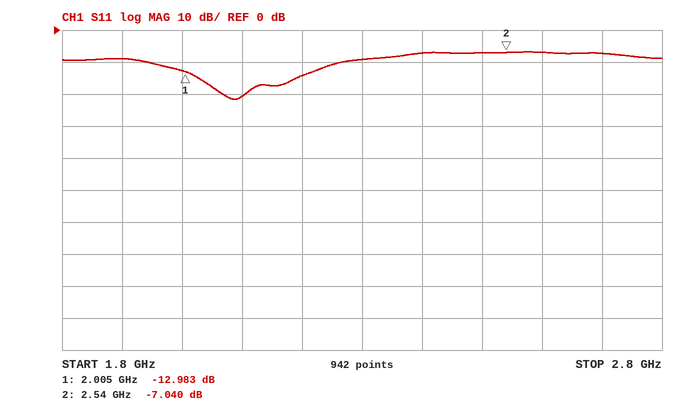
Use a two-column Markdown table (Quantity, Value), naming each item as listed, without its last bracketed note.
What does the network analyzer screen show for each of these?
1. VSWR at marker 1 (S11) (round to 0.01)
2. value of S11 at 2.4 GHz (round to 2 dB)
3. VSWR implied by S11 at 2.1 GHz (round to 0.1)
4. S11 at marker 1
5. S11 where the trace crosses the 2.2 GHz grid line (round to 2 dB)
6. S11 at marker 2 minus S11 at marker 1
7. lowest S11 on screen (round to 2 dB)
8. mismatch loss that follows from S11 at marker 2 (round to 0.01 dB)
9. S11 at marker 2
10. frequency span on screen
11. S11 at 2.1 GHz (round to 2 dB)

| Quantity | Value |
|---|---|
| VSWR at marker 1 (S11) | 1.58 |
| value of S11 at 2.4 GHz | -8 dB |
| VSWR implied by S11 at 2.1 GHz | 1.2 |
| S11 at marker 1 | -12.983 dB |
| S11 where the trace crosses the 2.2 GHz grid line | -14 dB |
| S11 at marker 2 minus S11 at marker 1 | 5.943 dB |
| lowest S11 on screen | -22 dB |
| mismatch loss that follows from S11 at marker 2 | 0.96 dB |
| S11 at marker 2 | -7.040 dB |
| frequency span on screen | 1 GHz |
| S11 at 2.1 GHz | -20 dB |
